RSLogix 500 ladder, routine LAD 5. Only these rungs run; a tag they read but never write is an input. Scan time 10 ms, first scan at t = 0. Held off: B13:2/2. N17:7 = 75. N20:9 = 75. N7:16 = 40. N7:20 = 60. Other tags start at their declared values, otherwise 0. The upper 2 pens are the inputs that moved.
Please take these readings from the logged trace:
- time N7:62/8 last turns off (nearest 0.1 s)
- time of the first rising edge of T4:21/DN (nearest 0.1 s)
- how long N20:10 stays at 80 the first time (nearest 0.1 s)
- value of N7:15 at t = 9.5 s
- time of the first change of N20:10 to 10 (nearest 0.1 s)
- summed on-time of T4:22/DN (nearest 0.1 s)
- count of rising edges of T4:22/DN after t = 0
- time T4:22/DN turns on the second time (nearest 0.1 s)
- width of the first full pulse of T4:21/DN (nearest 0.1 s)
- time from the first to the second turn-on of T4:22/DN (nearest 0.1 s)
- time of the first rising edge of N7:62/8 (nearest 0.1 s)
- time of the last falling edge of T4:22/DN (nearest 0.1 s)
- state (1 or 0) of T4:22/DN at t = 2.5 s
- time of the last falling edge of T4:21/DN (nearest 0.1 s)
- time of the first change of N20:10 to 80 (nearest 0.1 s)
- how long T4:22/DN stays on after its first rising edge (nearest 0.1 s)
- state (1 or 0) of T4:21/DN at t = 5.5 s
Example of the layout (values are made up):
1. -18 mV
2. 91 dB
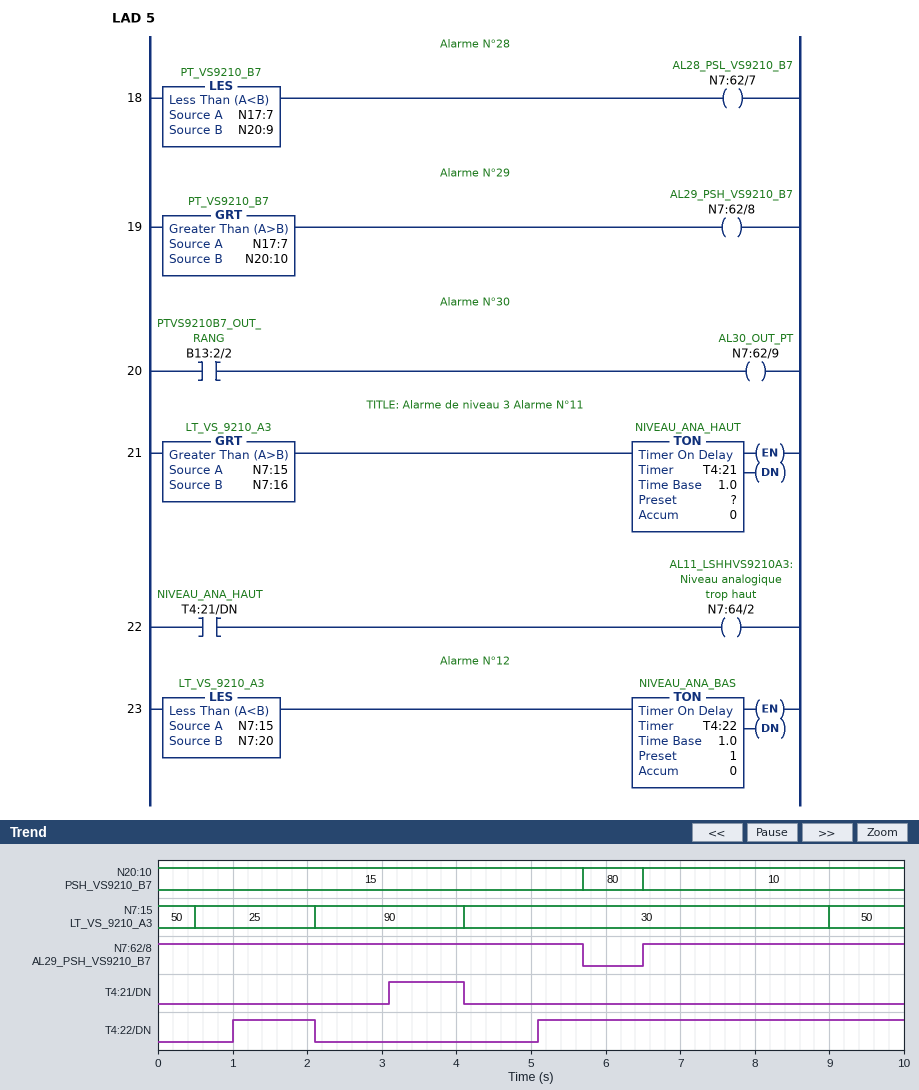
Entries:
1. 5.7 s
2. 3.1 s
3. 0.8 s
4. 50
5. 6.5 s
6. 6.0 s
7. 2
8. 5.1 s
9. 1.0 s
10. 4.1 s
11. 6.5 s
12. 2.1 s
13. 0
14. 4.1 s
15. 5.7 s
16. 1.1 s
17. 0
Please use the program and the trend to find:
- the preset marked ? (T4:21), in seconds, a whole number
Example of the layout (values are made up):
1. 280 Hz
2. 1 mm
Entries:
1. 1 s
